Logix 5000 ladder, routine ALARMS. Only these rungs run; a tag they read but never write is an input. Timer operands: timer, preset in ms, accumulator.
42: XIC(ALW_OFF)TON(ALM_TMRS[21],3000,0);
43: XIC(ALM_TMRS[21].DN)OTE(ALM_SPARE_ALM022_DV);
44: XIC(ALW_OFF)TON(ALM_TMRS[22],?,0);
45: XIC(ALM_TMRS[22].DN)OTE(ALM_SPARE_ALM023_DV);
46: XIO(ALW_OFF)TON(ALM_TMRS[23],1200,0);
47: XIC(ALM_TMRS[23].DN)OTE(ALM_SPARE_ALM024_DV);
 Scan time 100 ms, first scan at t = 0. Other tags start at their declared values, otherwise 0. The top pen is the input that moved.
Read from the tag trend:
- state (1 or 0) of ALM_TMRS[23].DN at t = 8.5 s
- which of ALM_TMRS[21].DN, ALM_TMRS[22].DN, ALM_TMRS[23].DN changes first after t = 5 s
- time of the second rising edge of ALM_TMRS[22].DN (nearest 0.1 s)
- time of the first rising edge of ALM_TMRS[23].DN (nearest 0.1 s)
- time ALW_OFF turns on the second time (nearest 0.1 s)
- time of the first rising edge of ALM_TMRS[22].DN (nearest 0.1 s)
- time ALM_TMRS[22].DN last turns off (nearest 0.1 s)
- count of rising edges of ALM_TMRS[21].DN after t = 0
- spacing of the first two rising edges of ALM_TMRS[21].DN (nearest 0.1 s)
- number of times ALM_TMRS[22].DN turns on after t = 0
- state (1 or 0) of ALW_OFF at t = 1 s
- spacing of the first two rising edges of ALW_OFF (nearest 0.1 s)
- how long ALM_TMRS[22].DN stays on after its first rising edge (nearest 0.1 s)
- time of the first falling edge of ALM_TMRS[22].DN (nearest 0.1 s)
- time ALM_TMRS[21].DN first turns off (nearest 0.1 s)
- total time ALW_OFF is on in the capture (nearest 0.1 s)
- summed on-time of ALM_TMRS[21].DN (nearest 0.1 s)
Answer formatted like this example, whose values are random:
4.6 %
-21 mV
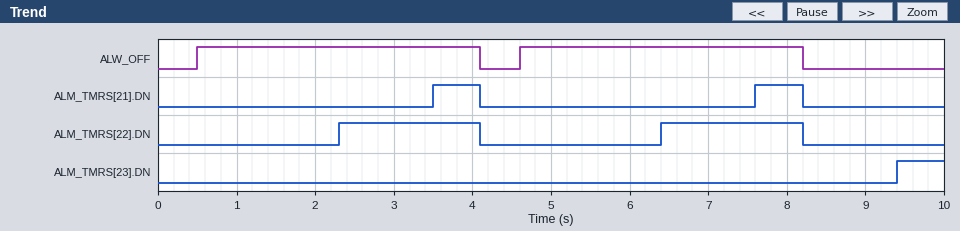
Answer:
0
ALM_TMRS[22].DN
6.4 s
9.4 s
4.6 s
2.3 s
8.2 s
2
4.1 s
2
1
4.1 s
1.8 s
4.1 s
4.1 s
7.2 s
1.2 s
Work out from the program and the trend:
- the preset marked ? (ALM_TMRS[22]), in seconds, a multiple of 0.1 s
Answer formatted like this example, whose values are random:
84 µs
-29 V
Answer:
1.8 s
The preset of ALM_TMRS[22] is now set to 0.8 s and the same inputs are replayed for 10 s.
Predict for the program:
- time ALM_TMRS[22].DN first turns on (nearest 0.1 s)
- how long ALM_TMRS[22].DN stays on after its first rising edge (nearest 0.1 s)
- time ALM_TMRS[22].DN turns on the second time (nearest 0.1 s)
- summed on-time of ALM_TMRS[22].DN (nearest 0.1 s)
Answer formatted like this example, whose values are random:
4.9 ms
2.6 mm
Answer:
1.3 s
2.8 s
5.4 s
5.6 s
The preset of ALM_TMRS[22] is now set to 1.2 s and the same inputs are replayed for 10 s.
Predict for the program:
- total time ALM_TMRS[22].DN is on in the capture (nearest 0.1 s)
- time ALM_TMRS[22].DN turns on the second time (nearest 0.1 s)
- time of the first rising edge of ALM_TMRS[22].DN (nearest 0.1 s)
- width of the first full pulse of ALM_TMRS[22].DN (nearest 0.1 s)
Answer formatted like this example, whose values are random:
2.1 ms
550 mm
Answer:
4.8 s
5.8 s
1.7 s
2.4 s
